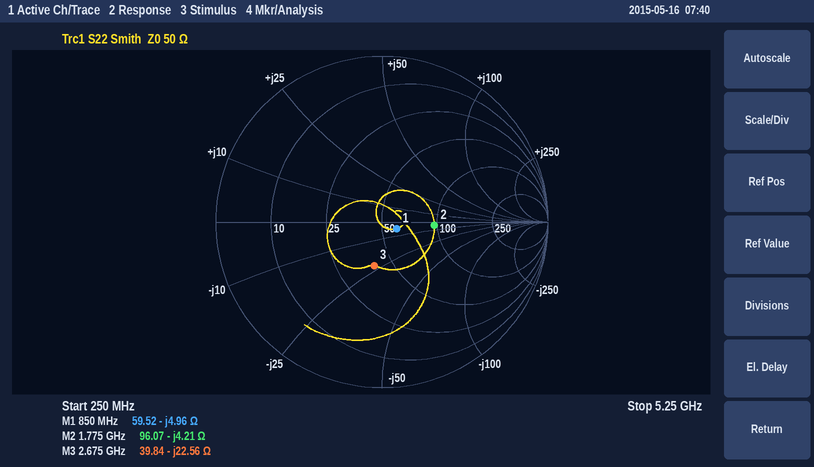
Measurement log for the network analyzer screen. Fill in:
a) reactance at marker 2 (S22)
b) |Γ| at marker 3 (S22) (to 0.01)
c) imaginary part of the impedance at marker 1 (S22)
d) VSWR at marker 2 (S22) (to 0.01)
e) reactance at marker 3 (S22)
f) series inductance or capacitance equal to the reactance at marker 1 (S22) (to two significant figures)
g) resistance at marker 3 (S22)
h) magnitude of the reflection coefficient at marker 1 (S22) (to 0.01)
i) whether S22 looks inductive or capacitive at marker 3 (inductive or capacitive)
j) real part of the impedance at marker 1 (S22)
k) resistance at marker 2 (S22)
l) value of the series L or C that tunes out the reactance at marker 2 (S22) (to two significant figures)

-4.21 Ω
0.27
-4.96 Ω
1.93
-22.56 Ω
38 pF
39.84 Ω
0.10
capacitive
59.52 Ω
96.07 Ω
380 pH
